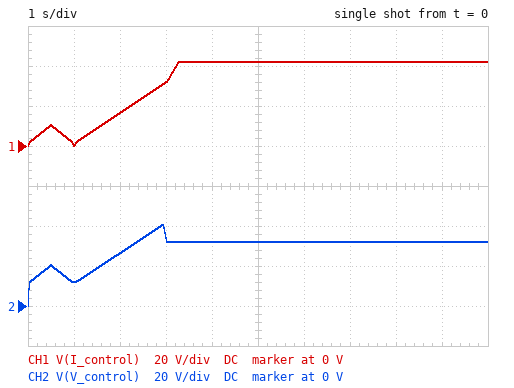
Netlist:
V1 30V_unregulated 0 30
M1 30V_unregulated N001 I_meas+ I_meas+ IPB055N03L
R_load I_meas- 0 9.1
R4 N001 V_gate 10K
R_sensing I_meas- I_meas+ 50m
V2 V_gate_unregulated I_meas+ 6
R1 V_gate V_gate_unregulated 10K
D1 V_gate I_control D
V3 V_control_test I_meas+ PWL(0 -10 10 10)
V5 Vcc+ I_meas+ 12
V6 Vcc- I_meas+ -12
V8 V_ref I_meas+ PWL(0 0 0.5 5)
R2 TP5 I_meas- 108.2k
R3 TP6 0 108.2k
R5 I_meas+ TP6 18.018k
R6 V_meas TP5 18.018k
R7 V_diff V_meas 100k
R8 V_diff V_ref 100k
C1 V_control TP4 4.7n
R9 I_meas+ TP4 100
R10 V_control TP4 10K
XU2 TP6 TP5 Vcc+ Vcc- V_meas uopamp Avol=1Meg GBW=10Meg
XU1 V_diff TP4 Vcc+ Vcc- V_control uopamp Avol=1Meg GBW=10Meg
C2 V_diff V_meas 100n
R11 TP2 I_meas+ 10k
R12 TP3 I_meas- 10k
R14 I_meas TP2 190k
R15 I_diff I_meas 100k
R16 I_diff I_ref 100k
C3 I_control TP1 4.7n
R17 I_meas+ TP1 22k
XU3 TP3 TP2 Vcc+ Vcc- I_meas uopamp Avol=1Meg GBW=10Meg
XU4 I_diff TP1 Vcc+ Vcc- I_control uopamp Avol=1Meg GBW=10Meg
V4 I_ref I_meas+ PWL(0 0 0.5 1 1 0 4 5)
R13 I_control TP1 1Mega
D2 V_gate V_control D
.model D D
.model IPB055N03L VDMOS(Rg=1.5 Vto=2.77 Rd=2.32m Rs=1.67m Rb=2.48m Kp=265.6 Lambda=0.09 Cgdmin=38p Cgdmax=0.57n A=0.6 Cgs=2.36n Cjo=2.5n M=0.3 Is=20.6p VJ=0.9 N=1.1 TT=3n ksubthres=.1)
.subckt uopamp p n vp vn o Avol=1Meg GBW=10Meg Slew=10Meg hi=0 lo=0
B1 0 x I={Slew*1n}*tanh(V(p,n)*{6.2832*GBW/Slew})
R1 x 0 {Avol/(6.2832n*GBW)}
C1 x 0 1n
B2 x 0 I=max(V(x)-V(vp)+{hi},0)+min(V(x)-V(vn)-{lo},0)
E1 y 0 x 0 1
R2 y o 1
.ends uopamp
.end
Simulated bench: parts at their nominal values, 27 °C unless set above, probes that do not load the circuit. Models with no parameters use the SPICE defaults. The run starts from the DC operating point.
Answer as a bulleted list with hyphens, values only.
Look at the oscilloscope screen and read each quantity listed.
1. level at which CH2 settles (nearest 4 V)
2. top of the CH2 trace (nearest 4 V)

- 32 V
- 40 V
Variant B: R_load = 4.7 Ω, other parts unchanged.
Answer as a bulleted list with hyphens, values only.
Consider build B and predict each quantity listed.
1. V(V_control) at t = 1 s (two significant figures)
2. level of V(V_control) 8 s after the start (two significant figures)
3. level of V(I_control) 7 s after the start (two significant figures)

- 12 V
- 35 V
- 26 V
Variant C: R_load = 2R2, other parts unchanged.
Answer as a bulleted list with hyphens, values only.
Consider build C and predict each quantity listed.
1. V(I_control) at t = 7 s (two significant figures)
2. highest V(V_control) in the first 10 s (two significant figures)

- 13 V
- 23 V
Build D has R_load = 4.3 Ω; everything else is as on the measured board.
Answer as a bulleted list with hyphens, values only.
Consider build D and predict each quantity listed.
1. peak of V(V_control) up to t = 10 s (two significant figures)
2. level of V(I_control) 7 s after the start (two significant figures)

- 33 V
- 24 V
